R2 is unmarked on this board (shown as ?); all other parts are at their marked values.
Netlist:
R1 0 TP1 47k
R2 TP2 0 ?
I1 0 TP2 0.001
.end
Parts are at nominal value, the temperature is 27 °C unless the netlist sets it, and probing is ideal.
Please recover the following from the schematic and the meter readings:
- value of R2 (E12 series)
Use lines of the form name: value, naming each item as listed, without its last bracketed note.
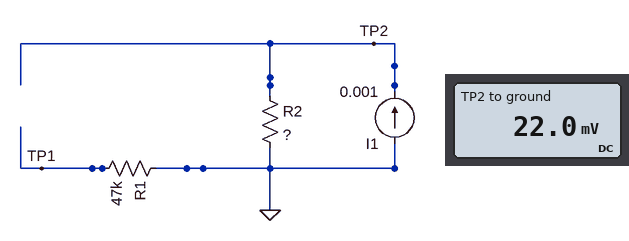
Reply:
value of R2: 22 Ω
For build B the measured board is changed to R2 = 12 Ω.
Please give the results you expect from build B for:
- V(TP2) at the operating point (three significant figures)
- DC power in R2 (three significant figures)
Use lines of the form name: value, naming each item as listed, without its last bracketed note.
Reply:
V(TP2) at the operating point: 12.0 mV
DC power in R2: 12.0 µW
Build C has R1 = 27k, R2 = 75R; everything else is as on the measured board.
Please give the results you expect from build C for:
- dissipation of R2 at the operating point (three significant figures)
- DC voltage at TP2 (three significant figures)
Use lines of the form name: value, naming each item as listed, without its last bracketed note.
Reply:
dissipation of R2 at the operating point: 75.0 µW
DC voltage at TP2: 75.0 mV
